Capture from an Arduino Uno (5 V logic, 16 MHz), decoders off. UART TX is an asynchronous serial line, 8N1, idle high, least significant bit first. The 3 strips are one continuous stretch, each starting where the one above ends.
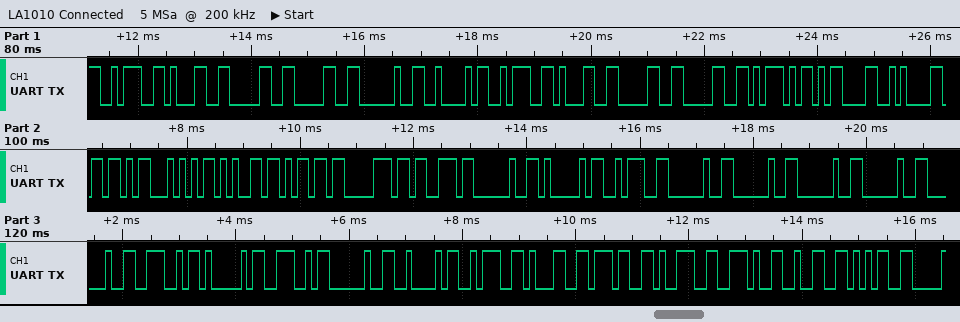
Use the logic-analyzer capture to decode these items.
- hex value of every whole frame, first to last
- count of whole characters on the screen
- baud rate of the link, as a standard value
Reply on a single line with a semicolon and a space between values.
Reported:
3A 31 30 30 20 42 3A 31 30 30 5D 0D 0A 5B 54 65 6D 70 73 20 41 3A 20 20 20 20 20 4E 41 4E 20 42 3A 31 37 39 2E 32 35; 39; 9600 baud
